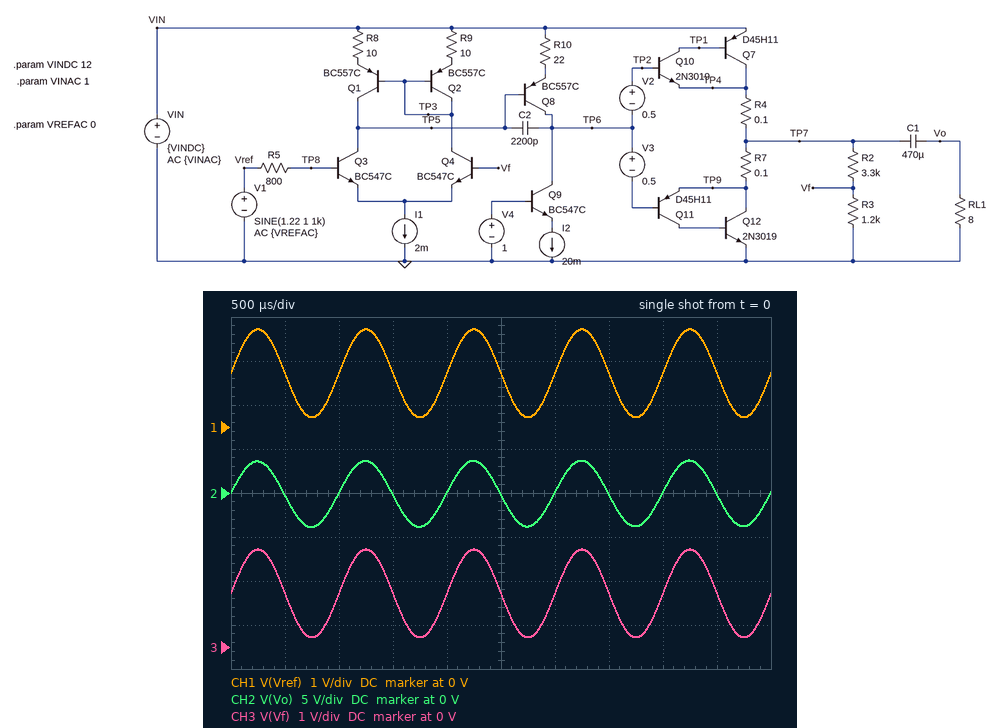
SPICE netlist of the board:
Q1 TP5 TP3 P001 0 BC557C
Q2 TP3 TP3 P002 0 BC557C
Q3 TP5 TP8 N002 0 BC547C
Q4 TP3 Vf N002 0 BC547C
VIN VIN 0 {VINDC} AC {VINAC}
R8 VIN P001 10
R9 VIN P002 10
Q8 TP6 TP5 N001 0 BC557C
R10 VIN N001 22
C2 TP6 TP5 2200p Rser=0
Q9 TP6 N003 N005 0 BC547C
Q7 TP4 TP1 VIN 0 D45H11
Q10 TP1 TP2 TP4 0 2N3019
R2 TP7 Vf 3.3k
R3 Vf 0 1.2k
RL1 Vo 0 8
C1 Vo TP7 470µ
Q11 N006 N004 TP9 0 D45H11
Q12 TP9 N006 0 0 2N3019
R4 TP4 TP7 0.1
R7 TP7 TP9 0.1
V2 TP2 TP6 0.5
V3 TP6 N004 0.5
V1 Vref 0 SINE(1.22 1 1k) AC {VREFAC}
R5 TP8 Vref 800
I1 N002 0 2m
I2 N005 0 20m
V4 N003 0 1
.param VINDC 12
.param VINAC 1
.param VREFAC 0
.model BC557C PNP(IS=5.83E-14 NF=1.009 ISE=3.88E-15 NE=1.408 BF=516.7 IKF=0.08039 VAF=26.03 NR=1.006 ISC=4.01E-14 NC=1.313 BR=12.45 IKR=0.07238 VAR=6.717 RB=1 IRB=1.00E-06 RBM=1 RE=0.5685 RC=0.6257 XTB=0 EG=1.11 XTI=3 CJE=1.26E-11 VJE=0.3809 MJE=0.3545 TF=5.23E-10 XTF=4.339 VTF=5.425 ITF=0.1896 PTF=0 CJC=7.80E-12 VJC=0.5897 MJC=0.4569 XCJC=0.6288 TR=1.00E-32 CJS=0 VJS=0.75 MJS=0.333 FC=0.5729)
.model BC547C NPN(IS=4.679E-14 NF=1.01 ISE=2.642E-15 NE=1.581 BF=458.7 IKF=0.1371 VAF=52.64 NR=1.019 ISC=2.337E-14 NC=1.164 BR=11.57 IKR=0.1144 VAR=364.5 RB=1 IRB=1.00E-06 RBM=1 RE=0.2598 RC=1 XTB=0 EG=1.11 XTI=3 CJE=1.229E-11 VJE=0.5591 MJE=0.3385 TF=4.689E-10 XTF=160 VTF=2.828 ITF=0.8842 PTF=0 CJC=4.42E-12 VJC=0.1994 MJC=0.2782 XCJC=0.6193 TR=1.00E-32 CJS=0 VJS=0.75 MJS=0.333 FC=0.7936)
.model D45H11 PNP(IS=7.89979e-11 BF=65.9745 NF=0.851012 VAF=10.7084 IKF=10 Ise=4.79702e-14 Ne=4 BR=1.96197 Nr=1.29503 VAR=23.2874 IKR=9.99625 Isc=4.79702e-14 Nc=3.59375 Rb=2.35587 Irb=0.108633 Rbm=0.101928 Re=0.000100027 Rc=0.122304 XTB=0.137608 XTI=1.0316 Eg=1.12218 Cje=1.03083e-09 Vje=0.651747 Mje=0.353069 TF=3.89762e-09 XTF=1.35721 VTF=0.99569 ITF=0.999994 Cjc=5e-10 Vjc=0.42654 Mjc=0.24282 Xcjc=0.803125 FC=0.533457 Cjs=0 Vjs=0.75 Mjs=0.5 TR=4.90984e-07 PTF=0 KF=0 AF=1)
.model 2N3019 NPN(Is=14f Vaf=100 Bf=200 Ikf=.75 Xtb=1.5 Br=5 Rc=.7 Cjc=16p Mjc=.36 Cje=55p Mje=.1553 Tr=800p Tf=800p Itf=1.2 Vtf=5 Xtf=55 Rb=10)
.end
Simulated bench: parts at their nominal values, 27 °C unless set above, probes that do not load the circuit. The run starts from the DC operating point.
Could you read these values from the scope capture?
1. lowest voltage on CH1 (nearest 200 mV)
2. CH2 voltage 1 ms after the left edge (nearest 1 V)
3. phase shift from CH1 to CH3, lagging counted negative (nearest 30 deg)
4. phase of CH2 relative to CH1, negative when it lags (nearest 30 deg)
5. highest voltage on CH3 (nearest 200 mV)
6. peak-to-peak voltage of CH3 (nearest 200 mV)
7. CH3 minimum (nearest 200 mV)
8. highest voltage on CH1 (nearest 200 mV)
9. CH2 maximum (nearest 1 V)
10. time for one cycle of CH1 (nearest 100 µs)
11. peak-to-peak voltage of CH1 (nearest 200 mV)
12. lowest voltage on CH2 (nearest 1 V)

200 mV
0 V
0 deg
0 deg
2.2 V
2.0 V
200 mV
2.2 V
4 V
1.0 ms
2.0 V
-4 V
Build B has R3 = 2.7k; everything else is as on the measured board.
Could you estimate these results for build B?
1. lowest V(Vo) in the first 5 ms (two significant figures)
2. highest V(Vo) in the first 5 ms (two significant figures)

-2.2 V
2.2 V
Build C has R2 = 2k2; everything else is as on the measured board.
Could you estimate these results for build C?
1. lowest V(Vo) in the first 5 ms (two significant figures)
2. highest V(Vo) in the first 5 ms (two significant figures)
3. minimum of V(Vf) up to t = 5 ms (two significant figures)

-2.9 V
2.8 V
230 mV
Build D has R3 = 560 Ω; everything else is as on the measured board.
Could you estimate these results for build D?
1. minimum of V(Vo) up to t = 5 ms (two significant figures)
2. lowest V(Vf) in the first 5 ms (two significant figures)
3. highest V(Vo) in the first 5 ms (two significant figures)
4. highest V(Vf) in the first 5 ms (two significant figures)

-6.9 V
220 mV
3.6 V
1.6 V
